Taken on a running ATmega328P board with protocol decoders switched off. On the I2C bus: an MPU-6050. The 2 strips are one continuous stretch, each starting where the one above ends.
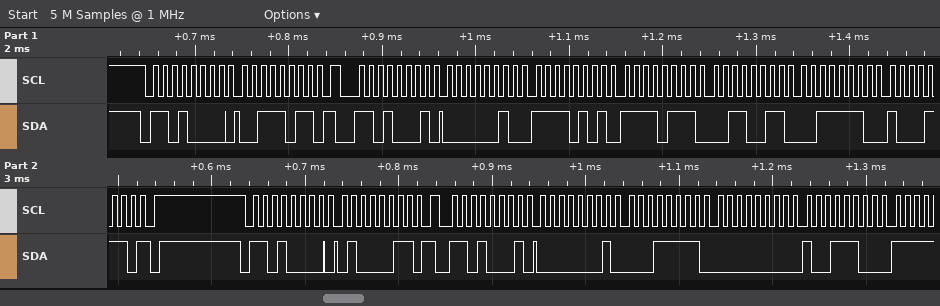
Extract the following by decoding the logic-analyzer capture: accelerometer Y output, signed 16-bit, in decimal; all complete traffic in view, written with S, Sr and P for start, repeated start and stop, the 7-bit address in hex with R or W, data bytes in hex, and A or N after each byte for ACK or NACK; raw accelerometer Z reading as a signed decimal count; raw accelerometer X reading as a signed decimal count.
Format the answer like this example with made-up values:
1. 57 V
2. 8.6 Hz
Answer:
1. -2253
2. S 68W A 3B A Sr 68R A 02 A F5 A F7 A 33 A 3E A 8E N P S 68W A 43 A Sr 68R A 01 A 1F A 00 A 9C A
3. 16014
4. 757
